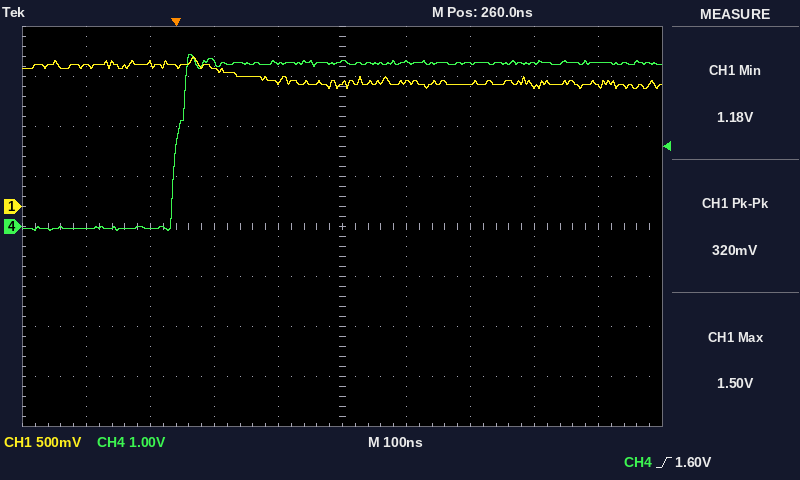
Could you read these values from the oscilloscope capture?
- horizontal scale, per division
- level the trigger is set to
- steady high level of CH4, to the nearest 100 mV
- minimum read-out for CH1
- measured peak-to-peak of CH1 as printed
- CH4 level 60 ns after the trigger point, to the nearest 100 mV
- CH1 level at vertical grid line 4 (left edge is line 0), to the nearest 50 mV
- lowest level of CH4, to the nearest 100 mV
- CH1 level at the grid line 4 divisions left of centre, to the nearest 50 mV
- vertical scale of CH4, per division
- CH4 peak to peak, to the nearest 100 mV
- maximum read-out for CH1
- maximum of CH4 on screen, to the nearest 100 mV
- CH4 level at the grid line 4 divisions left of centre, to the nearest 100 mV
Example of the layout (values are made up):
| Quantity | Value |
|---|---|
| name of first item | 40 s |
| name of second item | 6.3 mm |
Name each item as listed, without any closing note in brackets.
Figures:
| Quantity | Value |
|---|---|
| horizontal scale, per division | 100 ns |
| level the trigger is set to | 1.60 V |
| steady high level of CH4, to the nearest 100 mV | 3.3 V |
| minimum read-out for CH1 | 1.18 V |
| measured peak-to-peak of CH1 as printed | 320 mV |
| CH4 level 60 ns after the trigger point, to the nearest 100 mV | 3.3 V |
| CH1 level at vertical grid line 4 (left edge is line 0), to the nearest 50 mV | 1.25 V |
| lowest level of CH4, to the nearest 100 mV | -100 mV |
| CH1 level at the grid line 4 divisions left of centre, to the nearest 50 mV | 1.40 V |
| vertical scale of CH4, per division | 1 V |
| CH4 peak to peak, to the nearest 100 mV | 3.5 V |
| maximum read-out for CH1 | 1.50 V |
| maximum of CH4 on screen, to the nearest 100 mV | 3.4 V |
| CH4 level at the grid line 4 divisions left of centre, to the nearest 100 mV | 0.0 V |
